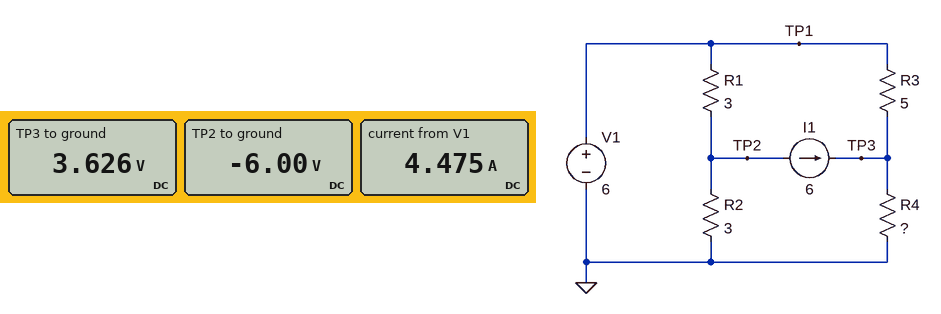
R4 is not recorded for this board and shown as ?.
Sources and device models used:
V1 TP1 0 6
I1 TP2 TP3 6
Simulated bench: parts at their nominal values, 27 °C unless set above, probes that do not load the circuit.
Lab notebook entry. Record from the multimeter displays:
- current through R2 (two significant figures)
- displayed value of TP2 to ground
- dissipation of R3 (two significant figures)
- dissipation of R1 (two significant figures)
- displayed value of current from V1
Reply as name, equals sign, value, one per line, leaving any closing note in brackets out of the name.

current through R2 = 2.0 A
displayed value of TP2 to ground = -6.00 V
dissipation of R3 = 1.1 W
dissipation of R1 = 48 W
displayed value of current from V1 = 4.475 A
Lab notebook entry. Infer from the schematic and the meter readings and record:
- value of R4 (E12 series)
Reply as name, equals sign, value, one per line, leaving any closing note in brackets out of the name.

value of R4 = 0.56 Ω
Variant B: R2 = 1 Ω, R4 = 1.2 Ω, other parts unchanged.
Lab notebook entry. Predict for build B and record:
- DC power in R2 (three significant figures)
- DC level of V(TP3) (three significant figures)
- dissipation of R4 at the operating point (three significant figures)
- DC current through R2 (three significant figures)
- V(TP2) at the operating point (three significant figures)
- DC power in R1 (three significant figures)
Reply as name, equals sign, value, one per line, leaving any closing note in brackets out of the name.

DC power in R2 = 9.00 W
DC level of V(TP3) = 6.97 V
dissipation of R4 at the operating point = 40.5 W
DC current through R2 = 3.00 A
V(TP2) at the operating point = -3.00 V
DC power in R1 = 27.0 W
